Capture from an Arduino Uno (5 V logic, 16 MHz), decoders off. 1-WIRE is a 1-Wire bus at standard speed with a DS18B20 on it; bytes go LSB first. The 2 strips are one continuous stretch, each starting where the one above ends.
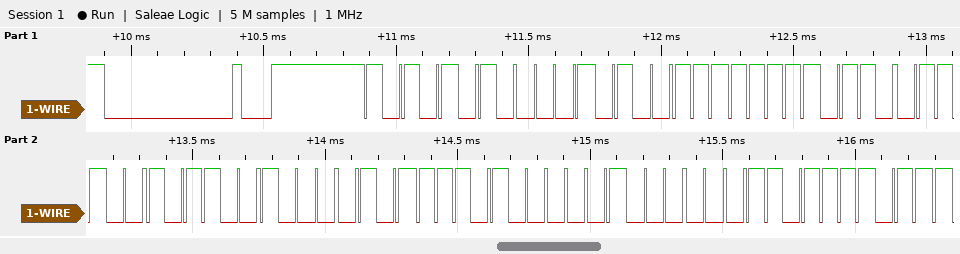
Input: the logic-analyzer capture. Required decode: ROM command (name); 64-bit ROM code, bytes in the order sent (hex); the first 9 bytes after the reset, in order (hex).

Match ROM
28 FF E6 34 A1 17 04 F6
55 28 FF E6 34 A1 17 04 F6
